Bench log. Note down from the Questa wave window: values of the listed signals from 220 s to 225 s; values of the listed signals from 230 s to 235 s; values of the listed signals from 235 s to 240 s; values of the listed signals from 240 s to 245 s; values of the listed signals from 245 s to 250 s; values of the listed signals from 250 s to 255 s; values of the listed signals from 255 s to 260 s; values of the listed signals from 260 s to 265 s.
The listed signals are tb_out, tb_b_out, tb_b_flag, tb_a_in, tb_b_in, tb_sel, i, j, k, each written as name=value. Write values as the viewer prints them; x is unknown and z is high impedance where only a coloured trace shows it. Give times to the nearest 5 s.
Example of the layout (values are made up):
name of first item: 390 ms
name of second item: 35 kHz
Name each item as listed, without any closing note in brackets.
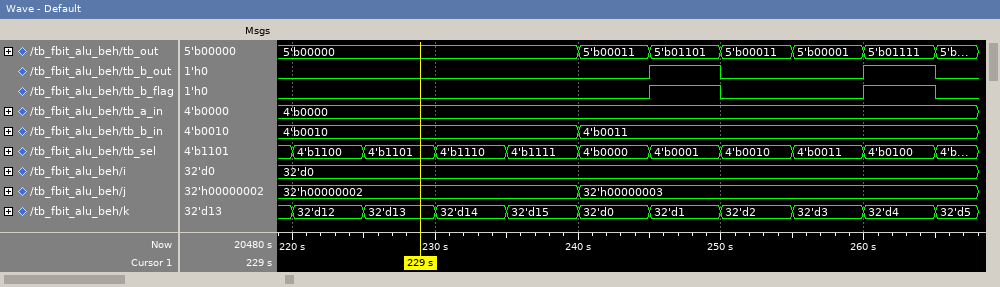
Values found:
values of the listed signals from 220 s to 225 s: tb_out=5'b00000, tb_b_out=0, tb_b_flag=0, tb_a_in=4'b0000, tb_b_in=4'b0010, tb_sel=4'b1100, i=32'd0, j=32'h00000002, k=32'd12
values of the listed signals from 230 s to 235 s: tb_out=5'b00000, tb_b_out=0, tb_b_flag=0, tb_a_in=4'b0000, tb_b_in=4'b0010, tb_sel=4'b1110, i=32'd0, j=32'h00000002, k=32'd14
values of the listed signals from 235 s to 240 s: tb_out=5'b00000, tb_b_out=0, tb_b_flag=0, tb_a_in=4'b0000, tb_b_in=4'b0010, tb_sel=4'b1111, i=32'd0, j=32'h00000002, k=32'd15
values of the listed signals from 240 s to 245 s: tb_out=5'b00011, tb_b_out=0, tb_b_flag=0, tb_a_in=4'b0000, tb_b_in=4'b0011, tb_sel=4'b0000, i=32'd0, j=32'h00000003, k=32'd0
values of the listed signals from 245 s to 250 s: tb_out=5'b01101, tb_b_out=1, tb_b_flag=1, tb_a_in=4'b0000, tb_b_in=4'b0011, tb_sel=4'b0001, i=32'd0, j=32'h00000003, k=32'd1
values of the listed signals from 250 s to 255 s: tb_out=5'b00011, tb_b_out=0, tb_b_flag=0, tb_a_in=4'b0000, tb_b_in=4'b0011, tb_sel=4'b0010, i=32'd0, j=32'h00000003, k=32'd2
values of the listed signals from 255 s to 260 s: tb_out=5'b00001, tb_b_out=0, tb_b_flag=0, tb_a_in=4'b0000, tb_b_in=4'b0011, tb_sel=4'b0011, i=32'd0, j=32'h00000003, k=32'd3
values of the listed signals from 260 s to 265 s: tb_out=5'b01111, tb_b_out=1, tb_b_flag=1, tb_a_in=4'b0000, tb_b_in=4'b0011, tb_sel=4'b0100, i=32'd0, j=32'h00000003, k=32'd4
